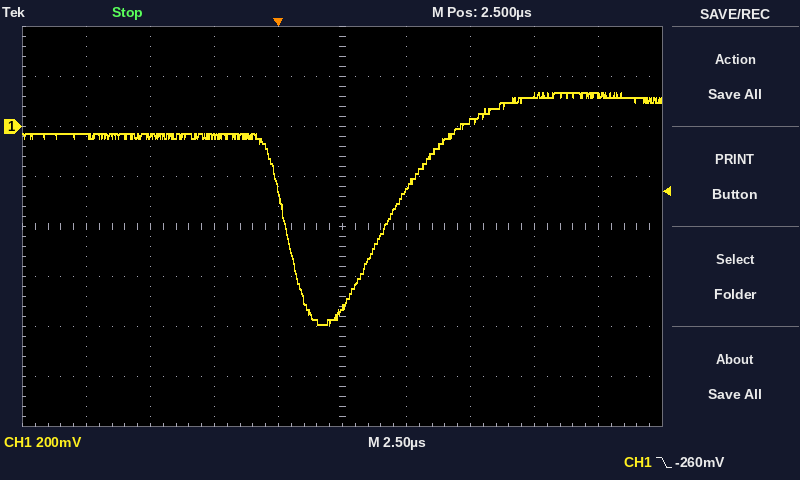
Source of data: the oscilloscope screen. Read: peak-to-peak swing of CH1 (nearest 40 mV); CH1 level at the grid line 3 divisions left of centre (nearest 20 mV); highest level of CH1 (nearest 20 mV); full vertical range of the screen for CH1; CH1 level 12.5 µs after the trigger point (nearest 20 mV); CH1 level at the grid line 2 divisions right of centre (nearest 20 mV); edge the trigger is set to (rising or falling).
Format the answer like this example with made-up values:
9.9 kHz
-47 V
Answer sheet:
920 mV
-40 mV
140 mV
1.6 V
120 mV
20 mV
falling
